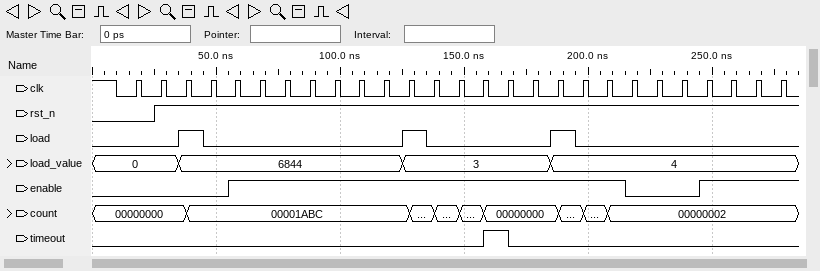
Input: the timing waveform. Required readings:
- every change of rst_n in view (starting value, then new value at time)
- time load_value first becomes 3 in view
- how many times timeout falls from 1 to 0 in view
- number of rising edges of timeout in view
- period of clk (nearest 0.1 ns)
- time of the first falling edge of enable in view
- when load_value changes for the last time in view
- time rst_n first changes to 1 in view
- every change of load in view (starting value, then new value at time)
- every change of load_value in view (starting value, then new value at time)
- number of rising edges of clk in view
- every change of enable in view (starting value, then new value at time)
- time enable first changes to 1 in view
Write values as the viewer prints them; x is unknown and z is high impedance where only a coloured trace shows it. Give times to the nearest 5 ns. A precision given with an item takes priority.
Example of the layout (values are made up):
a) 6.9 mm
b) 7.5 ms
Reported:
a) 0, 1 at 25 ns
b) 125 ns
c) 1
d) 1
e) 10 ns
f) 215 ns
g) 185 ns
h) 25 ns
i) 0, 1 at 35 ns, 0 at 45 ns, 1 at 125 ns, 0 at 135 ns, 1 at 185 ns, 0 at 195 ns
j) 0, 6844 at 35 ns, 3 at 125 ns, 4 at 185 ns
k) 27
l) 0, 1 at 55 ns, 0 at 215 ns, 1 at 245 ns
m) 55 ns
